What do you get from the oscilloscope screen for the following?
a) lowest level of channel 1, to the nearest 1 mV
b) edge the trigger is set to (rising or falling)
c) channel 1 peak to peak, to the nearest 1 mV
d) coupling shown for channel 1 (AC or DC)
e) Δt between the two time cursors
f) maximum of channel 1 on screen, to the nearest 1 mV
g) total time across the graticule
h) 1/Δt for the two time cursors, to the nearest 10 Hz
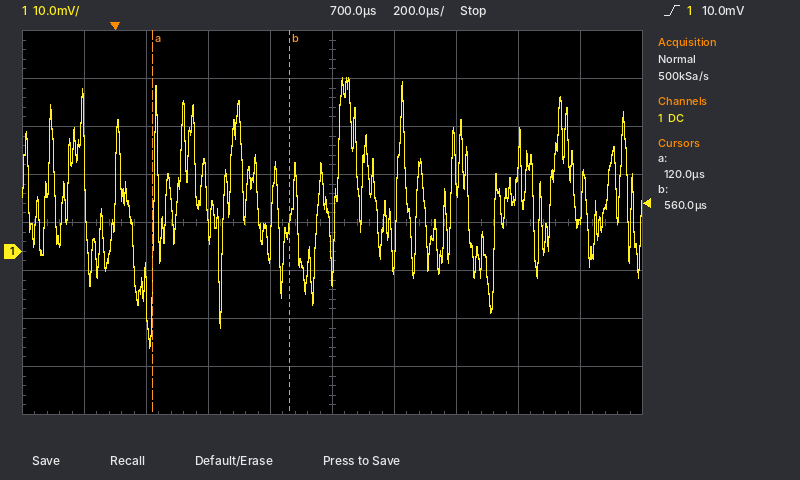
-20 mV
rising
56 mV
DC
440 µs
36 mV
2 ms
2.27 kHz
